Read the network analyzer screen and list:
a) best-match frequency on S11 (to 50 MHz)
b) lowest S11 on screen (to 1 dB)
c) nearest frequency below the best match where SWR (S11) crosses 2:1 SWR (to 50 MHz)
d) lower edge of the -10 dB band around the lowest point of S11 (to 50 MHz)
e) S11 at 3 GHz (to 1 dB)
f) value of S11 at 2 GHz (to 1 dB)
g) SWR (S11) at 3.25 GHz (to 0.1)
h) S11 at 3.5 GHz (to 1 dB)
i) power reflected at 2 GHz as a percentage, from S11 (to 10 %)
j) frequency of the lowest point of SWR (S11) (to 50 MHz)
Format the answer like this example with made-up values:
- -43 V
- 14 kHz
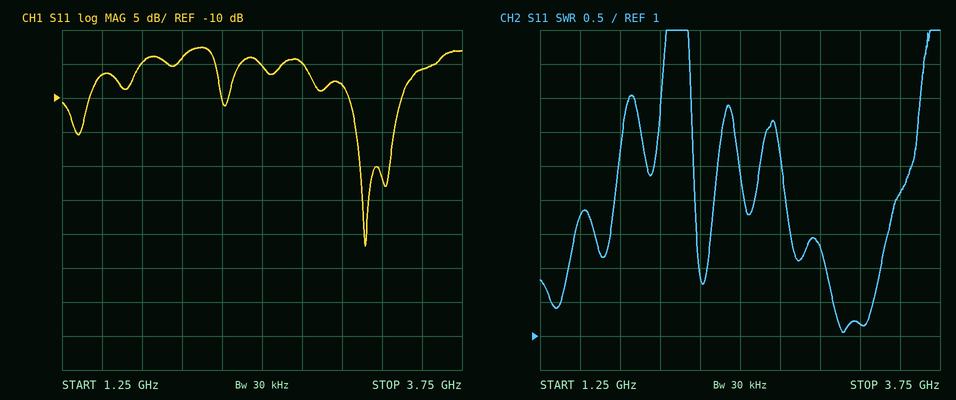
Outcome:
- 3.15 GHz
- -32 dB
- 3.05 GHz
- 3.05 GHz
- -8 dB
- -4 dB
- 1.2
- -6 dB
- 40 %
- 3.15 GHz
